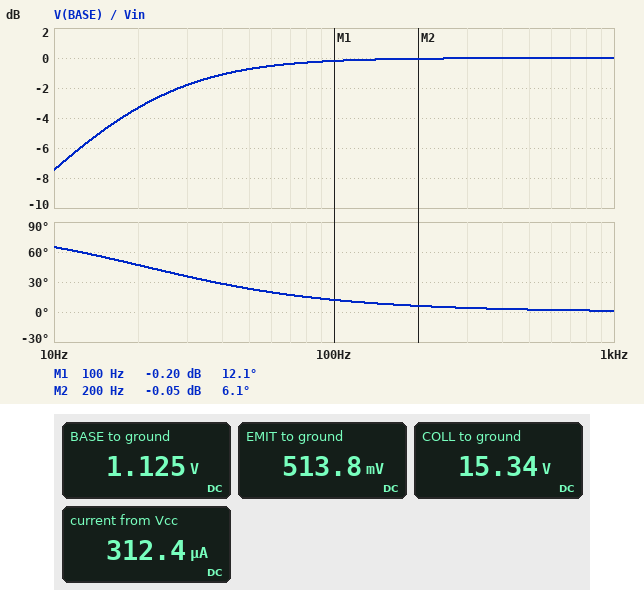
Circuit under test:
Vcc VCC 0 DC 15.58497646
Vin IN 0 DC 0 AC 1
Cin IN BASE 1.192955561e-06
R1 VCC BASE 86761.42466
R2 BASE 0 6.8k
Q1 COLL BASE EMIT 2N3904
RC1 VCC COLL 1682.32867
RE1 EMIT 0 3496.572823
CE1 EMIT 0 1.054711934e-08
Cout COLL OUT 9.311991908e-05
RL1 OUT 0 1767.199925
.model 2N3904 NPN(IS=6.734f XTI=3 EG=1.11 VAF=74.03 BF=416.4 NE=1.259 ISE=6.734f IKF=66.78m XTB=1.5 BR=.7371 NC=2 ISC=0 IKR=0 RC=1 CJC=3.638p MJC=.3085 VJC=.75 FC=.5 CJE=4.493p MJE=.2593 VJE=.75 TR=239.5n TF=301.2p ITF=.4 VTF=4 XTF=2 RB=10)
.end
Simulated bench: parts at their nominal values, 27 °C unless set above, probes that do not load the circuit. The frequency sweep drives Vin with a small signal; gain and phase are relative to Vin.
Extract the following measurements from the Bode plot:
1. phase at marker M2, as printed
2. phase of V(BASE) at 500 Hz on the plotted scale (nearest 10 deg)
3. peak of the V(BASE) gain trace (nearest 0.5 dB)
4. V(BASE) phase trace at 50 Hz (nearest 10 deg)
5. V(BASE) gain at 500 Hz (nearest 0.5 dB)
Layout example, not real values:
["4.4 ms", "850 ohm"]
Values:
["6.1 deg", "0 deg", "0 dB", "20 deg", "0 dB"]
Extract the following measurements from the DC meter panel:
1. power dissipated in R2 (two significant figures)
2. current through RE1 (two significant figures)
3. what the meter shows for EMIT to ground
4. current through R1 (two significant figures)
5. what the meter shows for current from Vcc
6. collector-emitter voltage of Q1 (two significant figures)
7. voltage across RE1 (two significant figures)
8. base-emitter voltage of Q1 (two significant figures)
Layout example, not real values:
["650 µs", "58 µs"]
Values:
["190 µW", "150 µA", "513.8 mV", "170 µA", "312.4 µA", "15 V", "510 mV", "610 mV"]
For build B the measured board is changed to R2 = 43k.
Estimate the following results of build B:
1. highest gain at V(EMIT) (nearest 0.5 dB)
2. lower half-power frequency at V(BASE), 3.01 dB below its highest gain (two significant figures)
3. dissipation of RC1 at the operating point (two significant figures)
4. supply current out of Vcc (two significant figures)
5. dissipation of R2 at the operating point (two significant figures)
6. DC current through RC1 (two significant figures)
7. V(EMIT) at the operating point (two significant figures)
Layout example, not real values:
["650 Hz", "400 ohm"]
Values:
["0 dB", "4.9 Hz", "2.5 mW", "1.3 mA", "570 µW", "1.2 mA", "4.3 V"]
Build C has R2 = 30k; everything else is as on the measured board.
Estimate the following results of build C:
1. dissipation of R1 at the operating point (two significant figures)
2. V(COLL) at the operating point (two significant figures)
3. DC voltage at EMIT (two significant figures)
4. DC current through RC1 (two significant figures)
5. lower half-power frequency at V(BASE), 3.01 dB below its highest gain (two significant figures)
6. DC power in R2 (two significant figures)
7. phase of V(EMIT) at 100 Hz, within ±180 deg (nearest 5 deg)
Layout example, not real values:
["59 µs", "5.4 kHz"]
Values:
["1.6 mW", "14 V", "3.2 V", "910 µA", "6.2 Hz", "500 µW", "5 deg"]
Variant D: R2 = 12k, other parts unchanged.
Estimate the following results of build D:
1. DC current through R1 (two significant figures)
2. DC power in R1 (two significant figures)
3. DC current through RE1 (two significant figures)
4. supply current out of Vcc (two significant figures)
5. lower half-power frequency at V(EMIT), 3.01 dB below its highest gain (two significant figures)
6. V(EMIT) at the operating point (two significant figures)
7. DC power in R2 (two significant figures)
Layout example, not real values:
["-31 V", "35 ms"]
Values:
["160 µA", "2.2 mW", "350 µA", "510 µA", "13 Hz", "1.2 V", "290 µW"]
